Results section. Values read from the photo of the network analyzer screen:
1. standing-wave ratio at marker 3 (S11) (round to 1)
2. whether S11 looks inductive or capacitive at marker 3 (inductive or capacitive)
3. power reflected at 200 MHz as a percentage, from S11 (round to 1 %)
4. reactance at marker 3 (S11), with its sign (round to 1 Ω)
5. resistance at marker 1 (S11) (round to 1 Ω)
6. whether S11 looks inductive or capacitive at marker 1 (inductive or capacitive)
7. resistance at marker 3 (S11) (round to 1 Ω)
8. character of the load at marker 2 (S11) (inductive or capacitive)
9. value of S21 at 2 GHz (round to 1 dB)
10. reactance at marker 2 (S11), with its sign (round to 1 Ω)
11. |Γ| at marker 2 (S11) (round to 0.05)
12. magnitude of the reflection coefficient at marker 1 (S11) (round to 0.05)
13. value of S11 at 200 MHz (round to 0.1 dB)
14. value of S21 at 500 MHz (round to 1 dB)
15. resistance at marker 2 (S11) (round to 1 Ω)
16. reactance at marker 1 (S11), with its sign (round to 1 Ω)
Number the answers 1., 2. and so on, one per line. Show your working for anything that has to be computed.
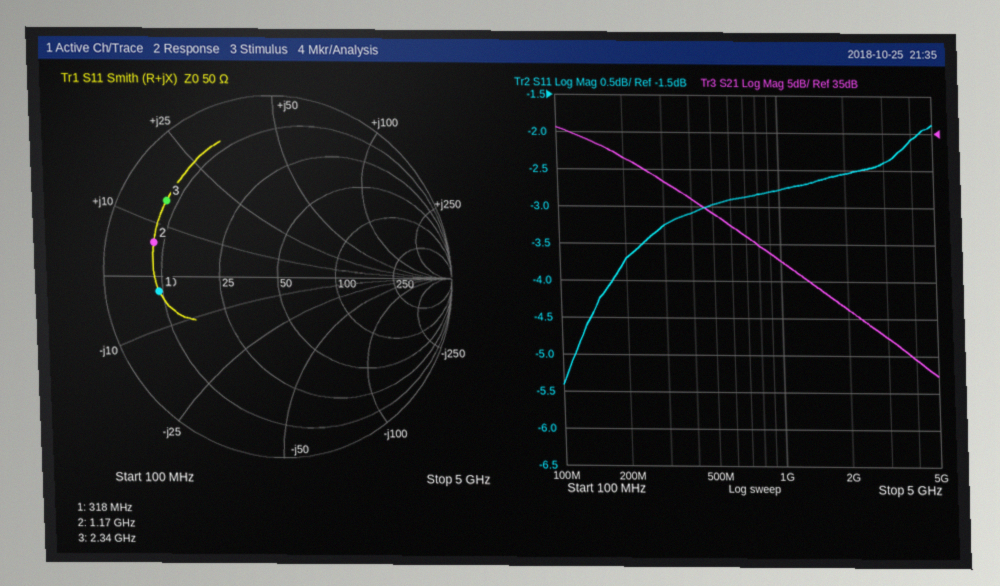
1. 7
2. inductive
3. 10^(-3.7/10) ≈ 43 %
4. +15 Ω
5. 9 Ω
6. capacitive
7. 8 Ω
8. inductive
9. 11 dB
10. +6 Ω
11. 0.75
12. 0.70
13. -3.7 dB
14. 24 dB
15. 8 Ω
16. -3 Ω
